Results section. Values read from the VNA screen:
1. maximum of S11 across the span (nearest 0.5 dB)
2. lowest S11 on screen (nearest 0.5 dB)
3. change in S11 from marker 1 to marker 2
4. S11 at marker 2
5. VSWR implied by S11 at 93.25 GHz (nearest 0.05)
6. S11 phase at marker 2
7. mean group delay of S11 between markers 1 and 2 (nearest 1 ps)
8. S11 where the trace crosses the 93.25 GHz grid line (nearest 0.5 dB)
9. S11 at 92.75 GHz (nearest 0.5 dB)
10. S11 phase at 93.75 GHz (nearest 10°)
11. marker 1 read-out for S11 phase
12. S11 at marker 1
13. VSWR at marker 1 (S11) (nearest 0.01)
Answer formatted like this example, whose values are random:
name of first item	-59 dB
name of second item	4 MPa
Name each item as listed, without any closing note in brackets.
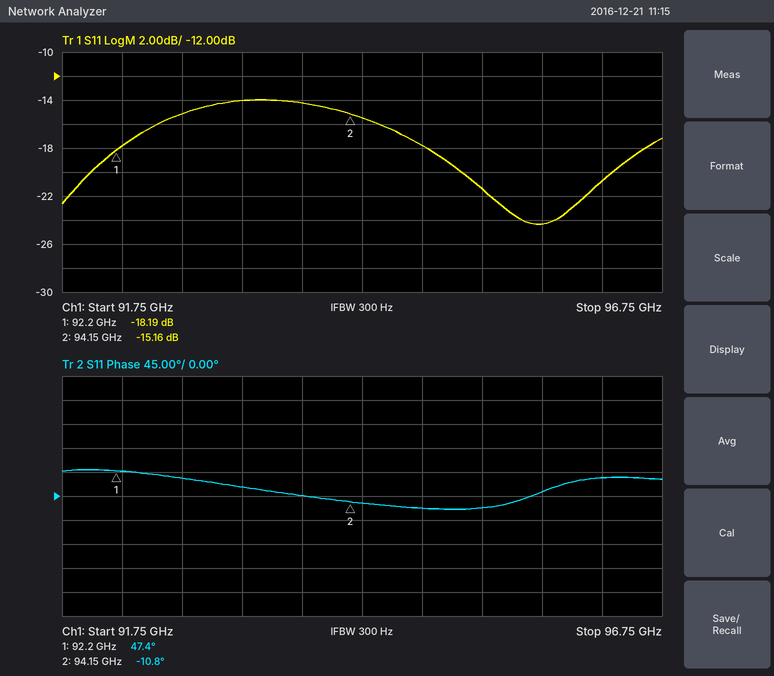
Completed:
maximum of S11 across the span	-14.0 dB
lowest S11 on screen	-24.5 dB
change in S11 from marker 1 to marker 2	3.03 dB
S11 at marker 2	-15.16 dB
VSWR implied by S11 at 93.25 GHz	1.50
S11 phase at marker 2	-10.8°
mean group delay of S11 between markers 1 and 2	83 ps
S11 where the trace crosses the 93.25 GHz grid line	-14.0 dB
S11 at 92.75 GHz	-15.0 dB
S11 phase at 93.75 GHz	0°
marker 1 read-out for S11 phase	47.4°
S11 at marker 1	-18.19 dB
VSWR at marker 1 (S11)	1.28
